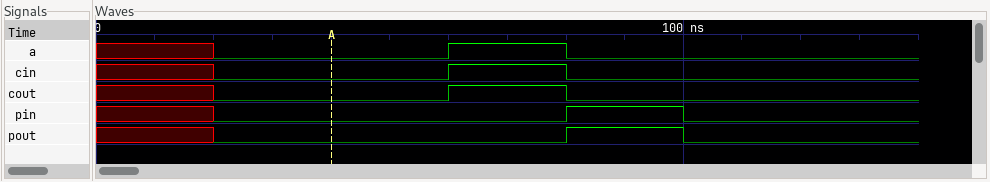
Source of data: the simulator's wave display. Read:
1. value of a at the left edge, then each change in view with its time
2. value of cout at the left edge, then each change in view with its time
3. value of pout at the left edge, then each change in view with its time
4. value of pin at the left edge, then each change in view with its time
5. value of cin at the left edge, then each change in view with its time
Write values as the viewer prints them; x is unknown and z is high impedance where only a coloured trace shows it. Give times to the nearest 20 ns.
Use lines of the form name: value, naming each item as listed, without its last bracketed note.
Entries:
value of a at the left edge, then each change in view with its time: x, 0 at 20 ns, 1 at 60 ns, 0 at 80 ns
value of cout at the left edge, then each change in view with its time: x, 0 at 20 ns, 1 at 60 ns, 0 at 80 ns
value of pout at the left edge, then each change in view with its time: x, 0 at 20 ns, 1 at 80 ns, 0 at 100 ns
value of pin at the left edge, then each change in view with its time: x, 0 at 20 ns, 1 at 80 ns, 0 at 100 ns
value of cin at the left edge, then each change in view with its time: x, 0 at 20 ns, 1 at 60 ns, 0 at 80 ns
